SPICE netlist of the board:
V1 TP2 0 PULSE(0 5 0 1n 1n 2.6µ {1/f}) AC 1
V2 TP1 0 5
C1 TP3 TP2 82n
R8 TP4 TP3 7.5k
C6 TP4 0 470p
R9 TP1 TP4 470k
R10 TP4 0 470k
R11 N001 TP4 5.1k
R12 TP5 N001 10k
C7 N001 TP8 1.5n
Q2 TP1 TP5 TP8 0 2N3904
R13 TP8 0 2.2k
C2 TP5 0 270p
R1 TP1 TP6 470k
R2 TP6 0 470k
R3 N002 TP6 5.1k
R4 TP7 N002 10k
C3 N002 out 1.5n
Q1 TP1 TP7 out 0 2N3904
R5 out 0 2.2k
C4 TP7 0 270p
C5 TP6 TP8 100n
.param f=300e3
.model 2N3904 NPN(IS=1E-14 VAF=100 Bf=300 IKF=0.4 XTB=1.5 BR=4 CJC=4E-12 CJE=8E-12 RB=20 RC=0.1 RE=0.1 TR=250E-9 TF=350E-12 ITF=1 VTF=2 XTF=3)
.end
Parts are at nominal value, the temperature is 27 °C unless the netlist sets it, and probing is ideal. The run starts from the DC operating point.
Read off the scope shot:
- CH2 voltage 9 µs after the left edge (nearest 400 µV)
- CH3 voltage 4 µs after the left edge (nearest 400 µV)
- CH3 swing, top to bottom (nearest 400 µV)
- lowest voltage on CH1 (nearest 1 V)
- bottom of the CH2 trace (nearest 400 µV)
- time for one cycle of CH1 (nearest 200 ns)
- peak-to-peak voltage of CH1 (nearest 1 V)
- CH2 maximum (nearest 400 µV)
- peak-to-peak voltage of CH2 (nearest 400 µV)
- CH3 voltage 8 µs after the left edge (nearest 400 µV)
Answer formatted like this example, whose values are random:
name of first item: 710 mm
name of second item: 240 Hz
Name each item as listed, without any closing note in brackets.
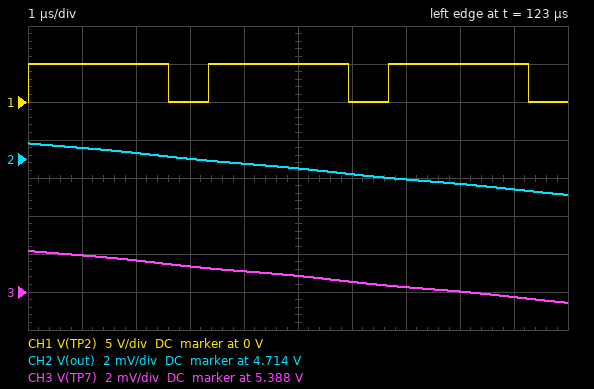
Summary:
CH2 voltage 9 µs after the left edge: 4.7124 V
CH3 voltage 4 µs after the left edge: 5.3892 V
CH3 swing, top to bottom: 2.8 mV
lowest voltage on CH1: 0 V
bottom of the CH2 trace: 4.7120 V
time for one cycle of CH1: 3.4 µs
peak-to-peak voltage of CH1: 5 V
CH2 maximum: 4.7148 V
peak-to-peak voltage of CH2: 2.8 mV
CH3 voltage 8 µs after the left edge: 5.3880 V
